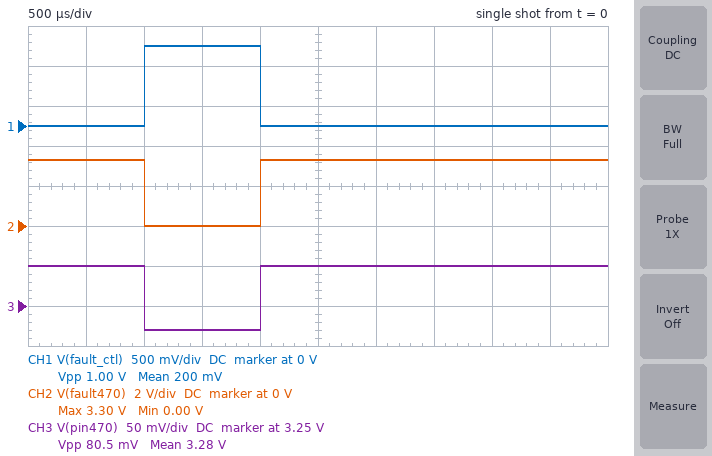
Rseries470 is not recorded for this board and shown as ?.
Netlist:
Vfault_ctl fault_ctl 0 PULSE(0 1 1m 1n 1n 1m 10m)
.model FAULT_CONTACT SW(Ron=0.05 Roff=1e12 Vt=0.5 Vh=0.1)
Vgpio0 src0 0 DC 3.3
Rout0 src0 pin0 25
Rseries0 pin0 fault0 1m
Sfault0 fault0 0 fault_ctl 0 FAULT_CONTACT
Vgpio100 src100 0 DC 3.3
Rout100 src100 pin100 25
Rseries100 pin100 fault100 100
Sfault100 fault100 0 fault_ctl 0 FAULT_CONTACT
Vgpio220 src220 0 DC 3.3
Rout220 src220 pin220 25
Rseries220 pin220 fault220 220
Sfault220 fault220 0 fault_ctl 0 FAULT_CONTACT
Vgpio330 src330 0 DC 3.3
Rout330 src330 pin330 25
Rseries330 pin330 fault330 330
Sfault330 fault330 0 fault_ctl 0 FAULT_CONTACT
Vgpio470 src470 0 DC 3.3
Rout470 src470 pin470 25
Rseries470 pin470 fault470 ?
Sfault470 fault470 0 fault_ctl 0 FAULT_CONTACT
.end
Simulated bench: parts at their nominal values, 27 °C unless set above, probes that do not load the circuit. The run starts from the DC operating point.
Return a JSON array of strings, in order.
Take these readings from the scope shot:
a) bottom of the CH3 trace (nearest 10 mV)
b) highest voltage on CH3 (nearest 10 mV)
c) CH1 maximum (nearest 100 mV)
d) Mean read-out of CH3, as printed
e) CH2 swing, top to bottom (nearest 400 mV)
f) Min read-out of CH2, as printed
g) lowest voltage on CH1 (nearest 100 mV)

["3.22 V", "3.30 V", "1.0 V", "3.28 V", "3.2 V", "0.00 V", "0 V"]
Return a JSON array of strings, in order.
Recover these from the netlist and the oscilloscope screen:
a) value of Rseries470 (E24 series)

["1 kΩ"]
